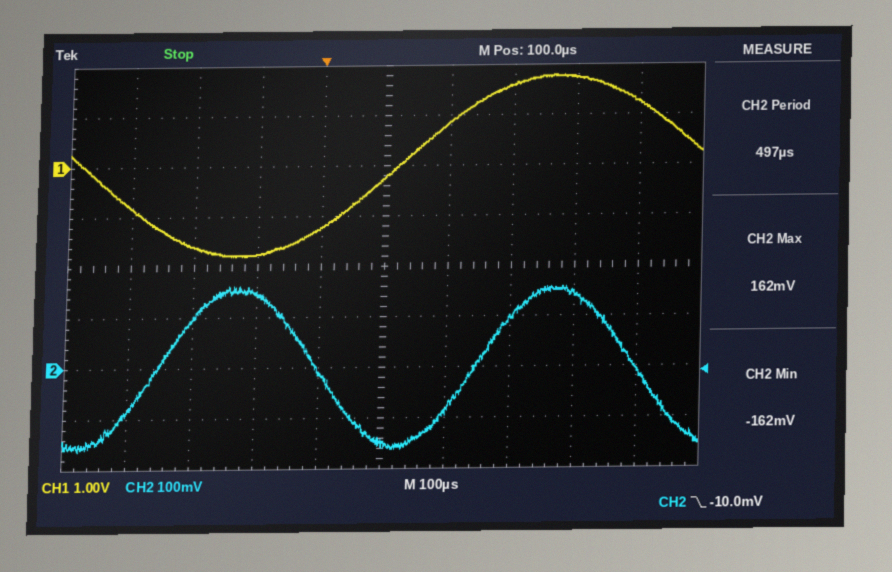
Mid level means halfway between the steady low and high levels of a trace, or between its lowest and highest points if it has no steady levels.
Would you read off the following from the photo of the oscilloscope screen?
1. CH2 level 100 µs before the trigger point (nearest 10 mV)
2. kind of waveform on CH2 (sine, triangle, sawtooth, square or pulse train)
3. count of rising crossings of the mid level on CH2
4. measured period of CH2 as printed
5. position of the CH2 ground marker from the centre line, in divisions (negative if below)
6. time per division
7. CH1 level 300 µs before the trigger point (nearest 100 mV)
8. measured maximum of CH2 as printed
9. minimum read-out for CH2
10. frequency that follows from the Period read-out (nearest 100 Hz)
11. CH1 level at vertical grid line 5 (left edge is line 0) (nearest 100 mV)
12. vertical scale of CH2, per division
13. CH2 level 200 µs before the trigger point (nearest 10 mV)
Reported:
150 mV
sine
2
497 µs
-2.0 div
100 µs
-800 mV
162 mV
-162 mV
2.0 kHz
-200 mV
100 mV
100 mV
